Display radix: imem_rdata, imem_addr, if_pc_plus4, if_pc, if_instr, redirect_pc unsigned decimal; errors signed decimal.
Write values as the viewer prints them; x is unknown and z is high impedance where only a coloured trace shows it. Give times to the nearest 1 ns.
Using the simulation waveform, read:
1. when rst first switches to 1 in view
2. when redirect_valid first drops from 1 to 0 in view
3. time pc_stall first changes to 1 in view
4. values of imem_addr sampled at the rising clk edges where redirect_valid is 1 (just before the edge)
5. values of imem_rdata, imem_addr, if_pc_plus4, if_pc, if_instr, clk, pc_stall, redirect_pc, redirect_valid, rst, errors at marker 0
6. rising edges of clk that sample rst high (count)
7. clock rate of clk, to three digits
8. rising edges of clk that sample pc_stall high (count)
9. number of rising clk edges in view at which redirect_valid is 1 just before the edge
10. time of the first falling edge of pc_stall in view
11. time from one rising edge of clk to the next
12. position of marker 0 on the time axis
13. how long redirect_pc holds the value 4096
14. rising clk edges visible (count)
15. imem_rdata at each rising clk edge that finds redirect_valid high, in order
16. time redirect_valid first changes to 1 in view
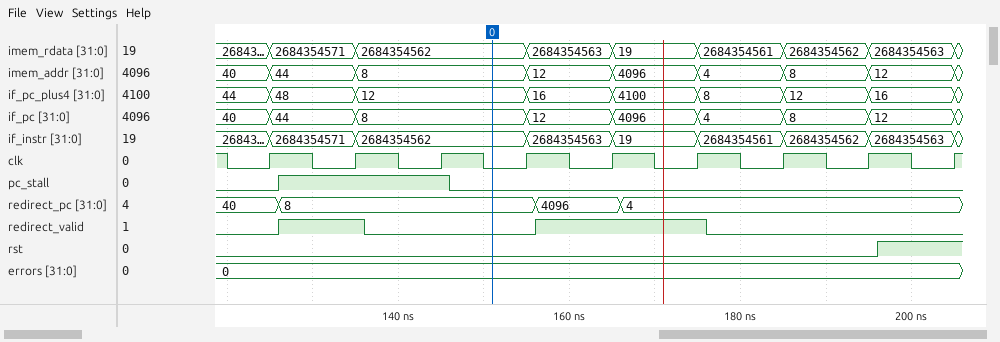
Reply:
196 ns
136 ns
126 ns
44, 12, 4096
imem_rdata=2684354562, imem_addr=8, if_pc_plus4=12, if_pc=8, if_instr=2684354562, clk=0, pc_stall=0, redirect_pc=8, redirect_valid=0, rst=0, errors=0
1
100 MHz
2
3
146 ns
10 ns
151 ns
10 ns
9
2684354571, 2684354563, 19
126 ns
